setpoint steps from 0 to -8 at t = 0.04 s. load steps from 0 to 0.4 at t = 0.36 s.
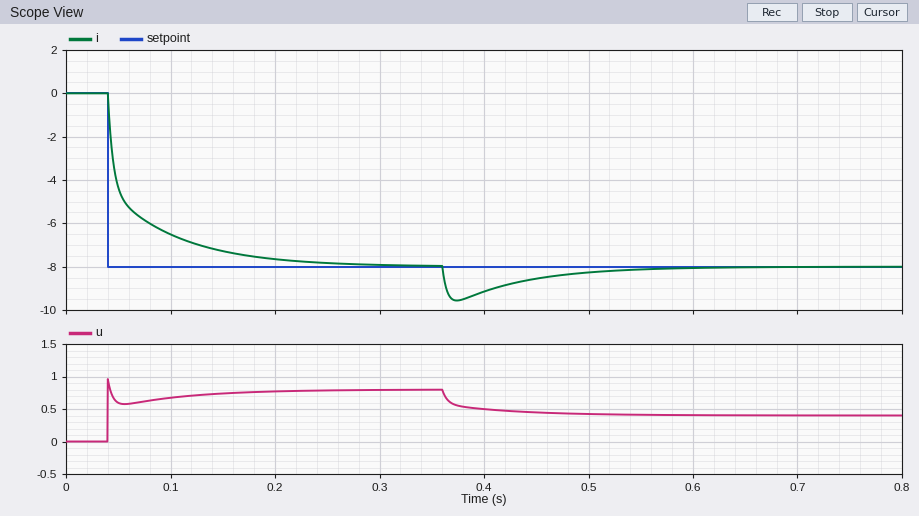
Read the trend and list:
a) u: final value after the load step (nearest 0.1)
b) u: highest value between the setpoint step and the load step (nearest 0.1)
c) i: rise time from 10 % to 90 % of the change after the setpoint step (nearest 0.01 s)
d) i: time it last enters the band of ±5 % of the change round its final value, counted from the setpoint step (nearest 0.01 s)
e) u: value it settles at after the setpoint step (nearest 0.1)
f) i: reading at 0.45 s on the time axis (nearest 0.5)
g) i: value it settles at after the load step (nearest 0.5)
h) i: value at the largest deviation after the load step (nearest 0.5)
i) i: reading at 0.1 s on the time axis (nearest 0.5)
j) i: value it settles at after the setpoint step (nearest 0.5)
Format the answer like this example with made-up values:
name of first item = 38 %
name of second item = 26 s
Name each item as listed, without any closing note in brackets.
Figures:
u: final value after the load step = 0.4
u: highest value between the setpoint step and the load step = 1.0
i: rise time from 10 % to 90 % of the change after the setpoint step = 0.10 s
i: time it last enters the band of ±5 % of the change round its final value, counted from the setpoint step = 0.15 s
u: value it settles at after the setpoint step = 0.8
i: reading at 0.45 s on the time axis = -8.5
i: value it settles at after the load step = -8.0
i: value at the largest deviation after the load step = -9.5
i: reading at 0.1 s on the time axis = -6.5
i: value it settles at after the setpoint step = -8.0
